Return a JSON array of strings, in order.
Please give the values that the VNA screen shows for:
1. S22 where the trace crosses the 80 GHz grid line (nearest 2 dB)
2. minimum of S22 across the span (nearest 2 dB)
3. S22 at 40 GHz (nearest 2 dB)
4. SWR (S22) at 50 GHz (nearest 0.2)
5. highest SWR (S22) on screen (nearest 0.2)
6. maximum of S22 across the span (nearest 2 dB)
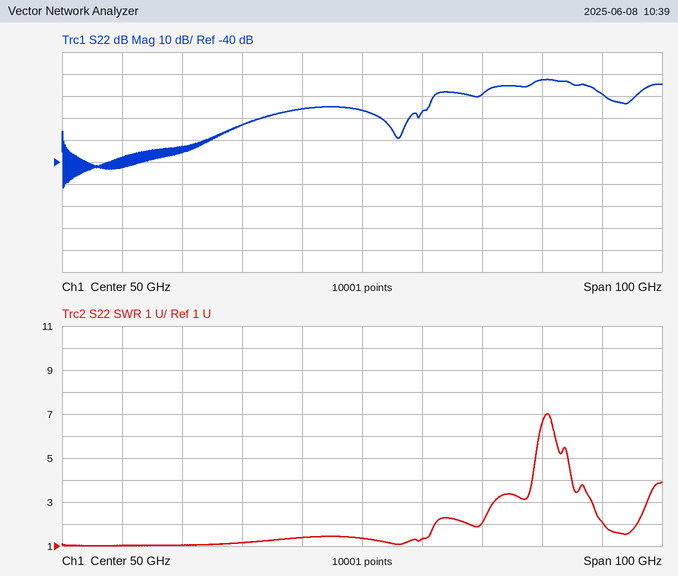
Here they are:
["-2 dB", "-52 dB", "-16 dB", "1.4", "7.0", "-2 dB"]
